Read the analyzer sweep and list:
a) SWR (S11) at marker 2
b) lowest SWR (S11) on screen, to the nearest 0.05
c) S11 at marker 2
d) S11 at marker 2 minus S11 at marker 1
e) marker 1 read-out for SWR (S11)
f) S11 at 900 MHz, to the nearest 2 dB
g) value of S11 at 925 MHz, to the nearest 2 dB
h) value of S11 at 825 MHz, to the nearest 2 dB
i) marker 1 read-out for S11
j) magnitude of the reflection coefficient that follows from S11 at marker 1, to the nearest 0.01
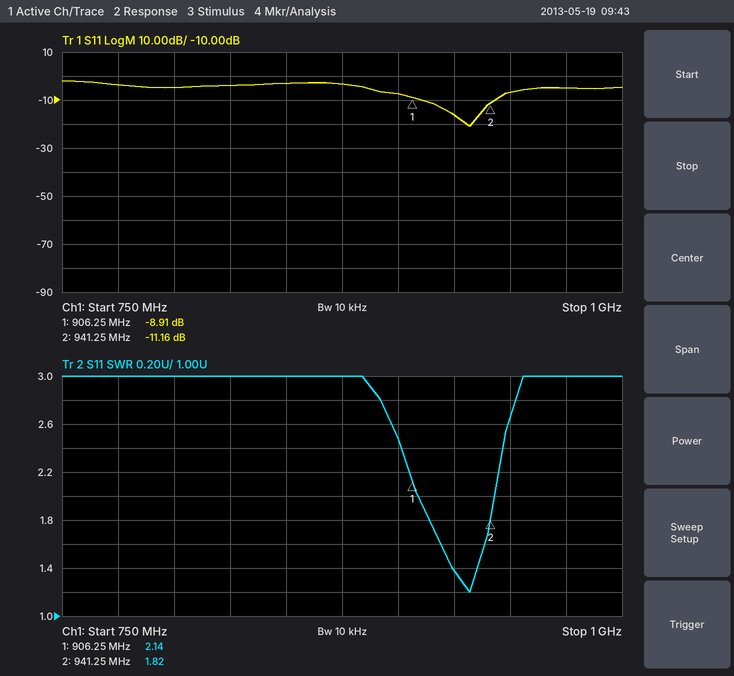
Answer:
1.82
1.20
-11.16 dB
-2.25 dB
2.14
-8 dB
-16 dB
-4 dB
-8.91 dB
0.36
